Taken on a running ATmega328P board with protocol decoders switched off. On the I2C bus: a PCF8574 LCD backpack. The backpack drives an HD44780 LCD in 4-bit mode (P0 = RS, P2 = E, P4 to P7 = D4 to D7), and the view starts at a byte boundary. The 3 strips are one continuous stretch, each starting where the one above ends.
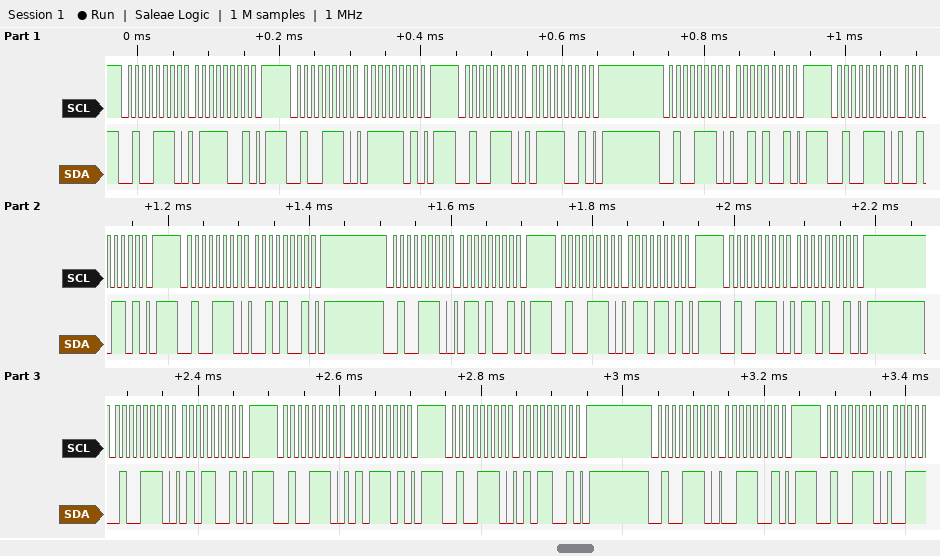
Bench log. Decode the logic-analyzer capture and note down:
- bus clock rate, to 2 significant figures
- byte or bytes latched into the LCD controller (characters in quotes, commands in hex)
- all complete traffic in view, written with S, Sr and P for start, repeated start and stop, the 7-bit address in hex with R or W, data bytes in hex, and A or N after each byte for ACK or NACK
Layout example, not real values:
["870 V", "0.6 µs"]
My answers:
["100 kHz", "'r' 'e'", "S 27W A 79 A P S 27W A 7D A P S 27W A 79 A P S 27W A 29 A P S 27W A 2D A P S 27W A 29 A P S 27W A 69 A P S 27W A 6D A P S 27W A 69 A P S 27W A 59 A P S 27W A 5D A P S 27W A 59 A P S 27W A 39 A P S 27W A"]
